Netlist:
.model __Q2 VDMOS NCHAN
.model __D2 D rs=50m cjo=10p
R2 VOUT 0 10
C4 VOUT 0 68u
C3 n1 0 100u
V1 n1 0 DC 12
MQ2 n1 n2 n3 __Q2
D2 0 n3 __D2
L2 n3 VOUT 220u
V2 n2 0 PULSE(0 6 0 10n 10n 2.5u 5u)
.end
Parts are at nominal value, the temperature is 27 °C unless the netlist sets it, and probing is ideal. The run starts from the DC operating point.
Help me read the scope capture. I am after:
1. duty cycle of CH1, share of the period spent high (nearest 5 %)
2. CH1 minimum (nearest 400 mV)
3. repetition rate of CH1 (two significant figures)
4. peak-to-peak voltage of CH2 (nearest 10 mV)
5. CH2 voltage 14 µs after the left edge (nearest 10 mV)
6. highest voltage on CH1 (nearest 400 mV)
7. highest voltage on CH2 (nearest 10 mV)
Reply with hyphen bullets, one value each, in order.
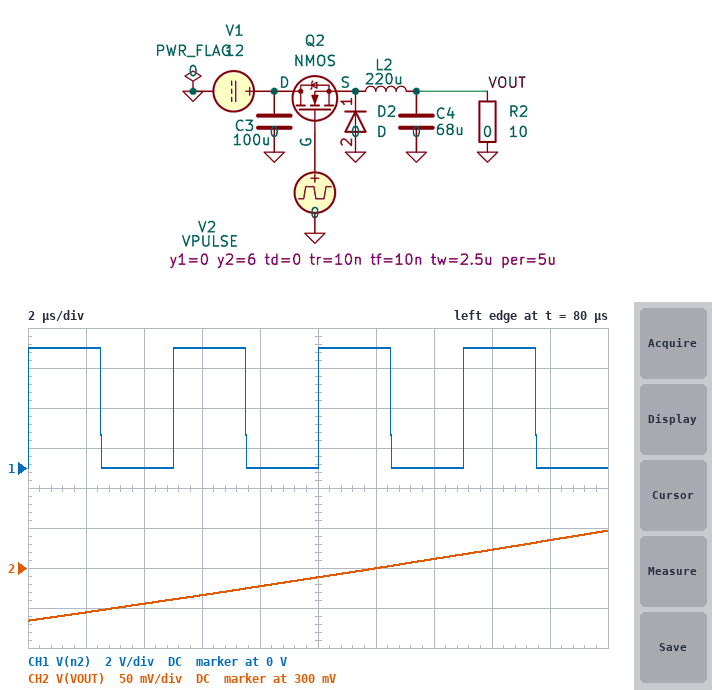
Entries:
- 50 %
- 0 V
- 200 kHz
- 110 mV
- 310 mV
- 6.0 V
- 350 mV
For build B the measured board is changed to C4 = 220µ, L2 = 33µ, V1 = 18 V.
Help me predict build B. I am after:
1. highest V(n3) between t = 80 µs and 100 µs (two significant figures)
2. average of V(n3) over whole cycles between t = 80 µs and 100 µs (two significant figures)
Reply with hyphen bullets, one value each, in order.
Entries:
- 2.7 V
- 850 mV
